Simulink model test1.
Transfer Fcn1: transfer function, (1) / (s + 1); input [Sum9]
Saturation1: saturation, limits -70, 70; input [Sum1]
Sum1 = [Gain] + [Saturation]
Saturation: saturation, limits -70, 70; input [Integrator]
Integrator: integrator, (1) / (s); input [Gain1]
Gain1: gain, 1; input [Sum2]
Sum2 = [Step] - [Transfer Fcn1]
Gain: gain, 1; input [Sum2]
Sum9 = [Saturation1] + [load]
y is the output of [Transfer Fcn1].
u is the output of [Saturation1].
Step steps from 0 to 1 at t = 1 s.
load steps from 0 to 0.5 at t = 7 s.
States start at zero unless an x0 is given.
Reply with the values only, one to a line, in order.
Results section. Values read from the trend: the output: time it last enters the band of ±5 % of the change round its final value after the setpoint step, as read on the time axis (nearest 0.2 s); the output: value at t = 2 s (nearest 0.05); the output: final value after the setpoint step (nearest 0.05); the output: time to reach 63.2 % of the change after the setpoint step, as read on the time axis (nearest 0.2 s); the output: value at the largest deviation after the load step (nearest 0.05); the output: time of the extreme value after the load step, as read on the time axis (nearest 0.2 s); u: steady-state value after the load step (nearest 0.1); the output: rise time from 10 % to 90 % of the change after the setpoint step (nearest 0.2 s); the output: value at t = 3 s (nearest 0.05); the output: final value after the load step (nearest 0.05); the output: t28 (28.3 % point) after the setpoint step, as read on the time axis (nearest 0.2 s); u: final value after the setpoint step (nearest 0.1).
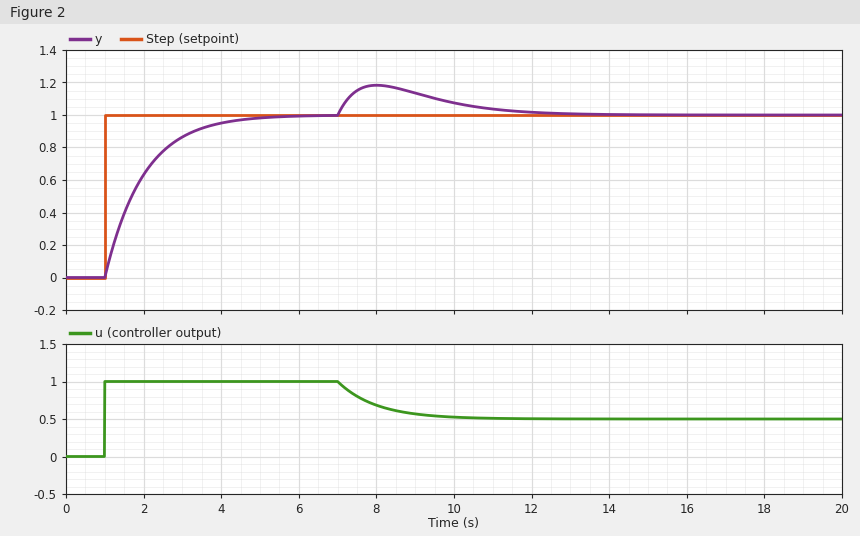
4.0 s
0.65
1.00
2.0 s
1.20
8.0 s
0.5
2.2 s
0.85
1.00
1.4 s
1.0
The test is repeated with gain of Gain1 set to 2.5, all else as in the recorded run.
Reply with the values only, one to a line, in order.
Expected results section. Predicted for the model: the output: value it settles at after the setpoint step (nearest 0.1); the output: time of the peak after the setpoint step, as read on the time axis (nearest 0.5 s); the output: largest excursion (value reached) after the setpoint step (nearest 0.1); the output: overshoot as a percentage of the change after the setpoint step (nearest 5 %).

1.0
3.0 s
1.1
10 %
